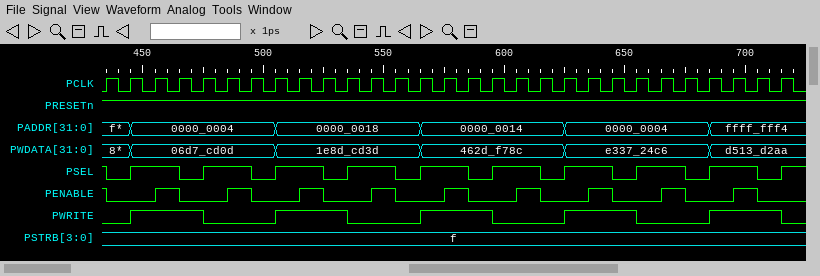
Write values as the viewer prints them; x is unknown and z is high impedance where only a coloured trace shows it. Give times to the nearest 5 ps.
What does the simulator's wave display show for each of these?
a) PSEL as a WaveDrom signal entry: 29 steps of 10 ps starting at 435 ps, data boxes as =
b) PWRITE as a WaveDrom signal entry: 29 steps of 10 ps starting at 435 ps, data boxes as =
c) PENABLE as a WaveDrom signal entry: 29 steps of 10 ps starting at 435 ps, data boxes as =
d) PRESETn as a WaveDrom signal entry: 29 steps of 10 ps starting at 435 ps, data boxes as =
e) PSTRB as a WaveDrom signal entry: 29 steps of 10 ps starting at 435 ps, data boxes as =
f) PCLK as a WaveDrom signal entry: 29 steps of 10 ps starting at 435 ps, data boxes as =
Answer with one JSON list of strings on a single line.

["{name: 'PSEL', wave: '01.01.01.01.01.01.01.01.01.01'}", "{name: 'PWRITE', wave: '01..0..1..0..1..0..1..0..1..0'}", "{name: 'PENABLE', wave: '0.10.10.10.10.10.10.10.10.10.'}", "{name: 'PRESETn', wave: '1............................'}", "{name: 'PSTRB', wave: '=............................', data: 'f'}", "{name: 'PCLK', wave: 'p............................'}"]
